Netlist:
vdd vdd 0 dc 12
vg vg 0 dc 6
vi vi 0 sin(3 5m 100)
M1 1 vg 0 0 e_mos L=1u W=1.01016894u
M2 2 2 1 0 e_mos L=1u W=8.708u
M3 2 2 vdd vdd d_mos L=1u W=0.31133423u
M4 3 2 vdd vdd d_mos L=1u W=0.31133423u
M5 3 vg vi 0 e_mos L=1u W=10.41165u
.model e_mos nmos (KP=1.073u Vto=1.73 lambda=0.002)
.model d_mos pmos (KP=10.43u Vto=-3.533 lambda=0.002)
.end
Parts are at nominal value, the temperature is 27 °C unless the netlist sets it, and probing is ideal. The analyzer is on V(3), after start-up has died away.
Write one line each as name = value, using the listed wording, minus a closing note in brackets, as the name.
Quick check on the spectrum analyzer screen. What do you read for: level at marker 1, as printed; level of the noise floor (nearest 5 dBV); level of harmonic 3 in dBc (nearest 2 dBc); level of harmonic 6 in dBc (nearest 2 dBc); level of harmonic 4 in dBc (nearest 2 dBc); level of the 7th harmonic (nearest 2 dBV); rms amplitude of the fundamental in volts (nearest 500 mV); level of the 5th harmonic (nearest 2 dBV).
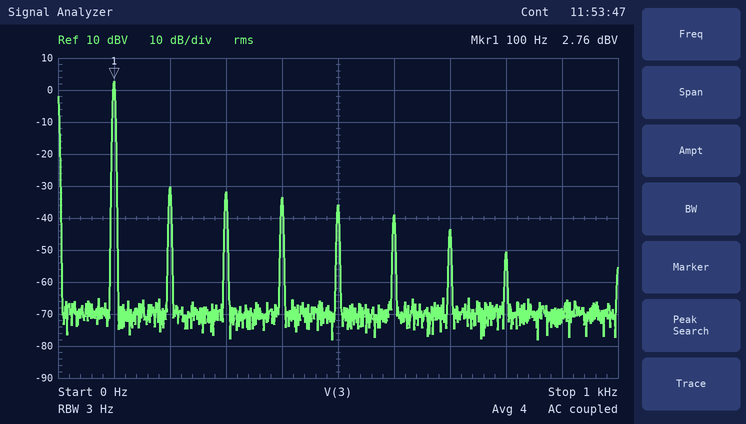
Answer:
level at marker 1, as printed = 2.76 dBV
level of the noise floor = -70 dBV
level of harmonic 3 in dBc = -34 dBc
level of harmonic 6 in dBc = -42 dBc
level of harmonic 4 in dBc = -36 dBc
level of the 7th harmonic = -44 dBV
rms amplitude of the fundamental in volts = 1.5 V
level of the 5th harmonic = -36 dBV
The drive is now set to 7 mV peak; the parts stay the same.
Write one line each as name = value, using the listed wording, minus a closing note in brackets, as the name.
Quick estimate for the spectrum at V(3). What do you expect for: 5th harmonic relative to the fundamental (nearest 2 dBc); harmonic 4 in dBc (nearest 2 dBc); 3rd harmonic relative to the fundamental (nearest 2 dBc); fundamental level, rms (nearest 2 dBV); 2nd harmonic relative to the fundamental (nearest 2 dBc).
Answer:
5th harmonic relative to the fundamental = -52 dBc
harmonic 4 in dBc = -30 dBc
3rd harmonic relative to the fundamental = -24 dBc
fundamental level, rms = 4 dBV
2nd harmonic relative to the fundamental = -20 dBc
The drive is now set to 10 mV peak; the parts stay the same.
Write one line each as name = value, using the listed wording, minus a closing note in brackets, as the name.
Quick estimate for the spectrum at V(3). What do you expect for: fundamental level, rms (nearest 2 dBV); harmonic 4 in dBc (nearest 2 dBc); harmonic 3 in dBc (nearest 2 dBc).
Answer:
fundamental level, rms = 6 dBV
harmonic 4 in dBc = -48 dBc
harmonic 3 in dBc = -20 dBc
